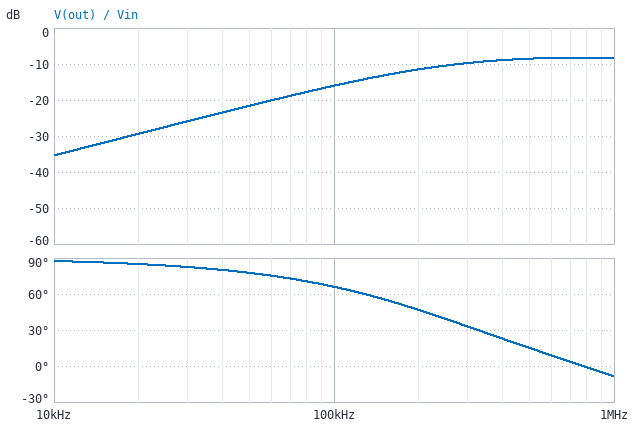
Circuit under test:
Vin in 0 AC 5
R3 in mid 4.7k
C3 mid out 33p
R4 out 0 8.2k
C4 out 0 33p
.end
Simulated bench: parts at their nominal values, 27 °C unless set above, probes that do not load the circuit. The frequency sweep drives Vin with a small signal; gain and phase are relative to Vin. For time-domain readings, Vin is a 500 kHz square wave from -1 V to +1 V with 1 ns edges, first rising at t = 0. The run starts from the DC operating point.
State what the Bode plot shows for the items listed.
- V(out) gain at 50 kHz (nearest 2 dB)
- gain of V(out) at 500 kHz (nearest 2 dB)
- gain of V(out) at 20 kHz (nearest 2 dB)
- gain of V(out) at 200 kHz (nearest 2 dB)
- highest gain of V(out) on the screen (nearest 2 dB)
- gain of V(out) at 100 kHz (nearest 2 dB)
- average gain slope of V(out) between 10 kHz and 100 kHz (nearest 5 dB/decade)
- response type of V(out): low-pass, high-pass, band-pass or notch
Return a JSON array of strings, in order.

["-22 dB", "-8 dB", "-30 dB", "-12 dB", "-8 dB", "-16 dB", "20 dB/decade", "high-pass"]
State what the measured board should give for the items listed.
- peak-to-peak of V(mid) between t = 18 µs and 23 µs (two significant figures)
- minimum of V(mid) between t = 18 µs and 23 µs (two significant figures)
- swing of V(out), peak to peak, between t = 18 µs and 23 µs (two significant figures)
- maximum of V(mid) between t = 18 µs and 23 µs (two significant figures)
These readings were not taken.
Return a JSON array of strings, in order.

["1.9 V", "-950 mV", "1.1 V", "950 mV"]
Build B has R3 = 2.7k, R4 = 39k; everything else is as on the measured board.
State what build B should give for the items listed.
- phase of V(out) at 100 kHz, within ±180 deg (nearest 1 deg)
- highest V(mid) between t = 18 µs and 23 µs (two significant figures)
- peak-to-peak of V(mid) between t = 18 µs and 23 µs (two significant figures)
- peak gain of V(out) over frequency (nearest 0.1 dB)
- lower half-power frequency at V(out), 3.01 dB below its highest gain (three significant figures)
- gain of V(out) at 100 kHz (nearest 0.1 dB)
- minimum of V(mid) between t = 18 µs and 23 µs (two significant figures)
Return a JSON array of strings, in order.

["30 deg", "990 mV", "2.0 V", "-6.3 dB", "58.8 kHz", "-7.5 dB", "-990 mV"]
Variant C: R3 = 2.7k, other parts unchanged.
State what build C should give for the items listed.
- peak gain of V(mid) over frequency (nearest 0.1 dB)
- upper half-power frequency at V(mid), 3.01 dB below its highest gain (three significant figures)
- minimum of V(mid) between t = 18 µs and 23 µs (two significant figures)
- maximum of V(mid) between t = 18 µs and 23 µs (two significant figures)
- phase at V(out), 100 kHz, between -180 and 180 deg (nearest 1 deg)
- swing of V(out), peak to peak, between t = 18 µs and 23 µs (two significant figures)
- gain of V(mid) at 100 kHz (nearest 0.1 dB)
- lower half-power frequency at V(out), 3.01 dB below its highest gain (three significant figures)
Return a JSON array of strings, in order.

["0 dB", "3.23 MHz", "-970 mV", "970 mV", "68 deg", "1.3 V", "-0.1 dB", "239 kHz"]
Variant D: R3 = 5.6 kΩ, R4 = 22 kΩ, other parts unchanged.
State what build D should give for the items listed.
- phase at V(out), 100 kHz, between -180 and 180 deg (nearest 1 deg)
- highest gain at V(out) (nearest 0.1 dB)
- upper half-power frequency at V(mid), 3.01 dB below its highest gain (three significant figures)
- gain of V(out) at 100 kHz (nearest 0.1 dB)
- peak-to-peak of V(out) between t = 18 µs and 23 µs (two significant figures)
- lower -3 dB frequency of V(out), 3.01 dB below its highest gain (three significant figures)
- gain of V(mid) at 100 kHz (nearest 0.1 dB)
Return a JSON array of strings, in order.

["43 deg", "-7.1 dB", "1.60 MHz", "-9.7 dB", "1.0 V", "92.8 kHz", "-0.3 dB"]
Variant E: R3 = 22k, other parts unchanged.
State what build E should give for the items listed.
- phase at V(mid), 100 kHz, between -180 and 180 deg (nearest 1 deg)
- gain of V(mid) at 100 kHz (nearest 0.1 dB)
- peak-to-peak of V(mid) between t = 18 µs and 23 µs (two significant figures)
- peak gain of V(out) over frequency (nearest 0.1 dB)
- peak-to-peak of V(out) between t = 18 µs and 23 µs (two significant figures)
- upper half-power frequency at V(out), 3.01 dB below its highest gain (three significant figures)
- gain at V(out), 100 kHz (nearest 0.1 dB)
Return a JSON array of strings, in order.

["-22 deg", "-1.2 dB", "1.3 V", "-13.4 dB", "470 mV", "1.14 MHz", "-17.1 dB"]
